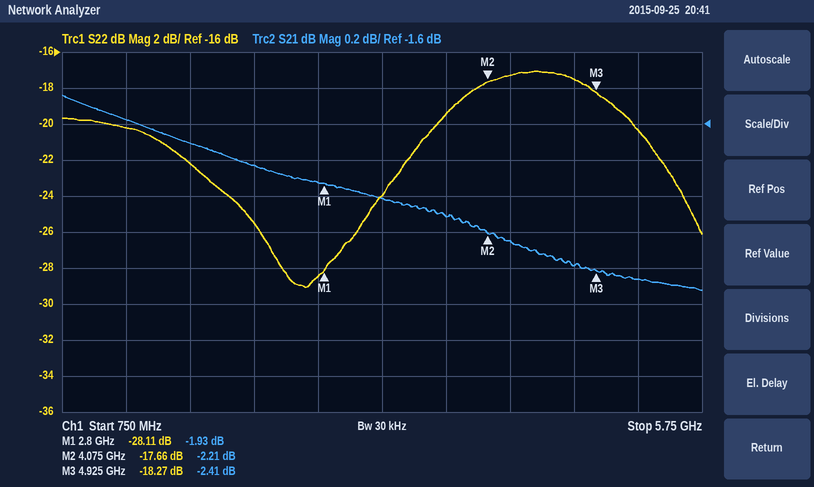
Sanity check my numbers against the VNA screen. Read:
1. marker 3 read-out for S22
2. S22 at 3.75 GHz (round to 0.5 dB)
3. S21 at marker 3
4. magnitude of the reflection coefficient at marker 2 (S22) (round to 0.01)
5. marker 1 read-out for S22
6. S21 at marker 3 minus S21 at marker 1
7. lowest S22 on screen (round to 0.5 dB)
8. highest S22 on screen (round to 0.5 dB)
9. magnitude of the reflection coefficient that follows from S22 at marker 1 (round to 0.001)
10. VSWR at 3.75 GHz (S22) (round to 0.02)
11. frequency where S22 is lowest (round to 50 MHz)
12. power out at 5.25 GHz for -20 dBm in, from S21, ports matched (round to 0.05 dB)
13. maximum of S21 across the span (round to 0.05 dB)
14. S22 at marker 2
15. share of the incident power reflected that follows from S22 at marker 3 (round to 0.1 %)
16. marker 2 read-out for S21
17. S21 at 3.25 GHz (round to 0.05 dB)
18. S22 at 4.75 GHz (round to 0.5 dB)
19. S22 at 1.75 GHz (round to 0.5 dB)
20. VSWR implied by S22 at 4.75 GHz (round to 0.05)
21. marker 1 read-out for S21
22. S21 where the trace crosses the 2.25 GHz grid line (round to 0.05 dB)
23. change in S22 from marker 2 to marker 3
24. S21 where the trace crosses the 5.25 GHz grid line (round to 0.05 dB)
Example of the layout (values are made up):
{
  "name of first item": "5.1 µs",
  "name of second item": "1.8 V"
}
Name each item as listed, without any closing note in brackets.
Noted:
{
  "marker 3 read-out for S22": "-18.27 dB",
  "S22 at 3.75 GHz": "-19.5 dB",
  "S21 at marker 3": "-2.41 dB",
  "magnitude of the reflection coefficient at marker 2 (S22)": "0.13",
  "marker 1 read-out for S22": "-28.11 dB",
  "S21 at marker 3 minus S21 at marker 1": "-0.48 dB",
  "lowest S22 on screen": "-29.0 dB",
  "highest S22 on screen": "-17.0 dB",
  "magnitude of the reflection coefficient that follows from S22 at marker 1": "0.039",
  "VSWR at 3.75 GHz (S22)": "1.24",
  "frequency where S22 is lowest": "2.65 GHz",
  "power out at 5.25 GHz for -20 dBm in, from S21, ports matched": "-22.45 dBm",
  "maximum of S21 across the span": "-1.45 dB",
  "S22 at marker 2": "-17.66 dB",
  "share of the incident power reflected that follows from S22 at marker 3": "1.5 %",
  "marker 2 read-out for S21": "-2.21 dB",
  "S21 at 3.25 GHz": "-2.00 dB",
  "S22 at 4.75 GHz": "-17.5 dB",
  "S22 at 1.75 GHz": "-22.0 dB",
  "VSWR implied by S22 at 4.75 GHz": "1.30",
  "marker 1 read-out for S21": "-1.93 dB",
  "S21 where the trace crosses the 2.25 GHz grid line": "-1.85 dB",
  "change in S22 from marker 2 to marker 3": "-0.61 dB",
  "S21 where the trace crosses the 5.25 GHz grid line": "-2.45 dB"
}
